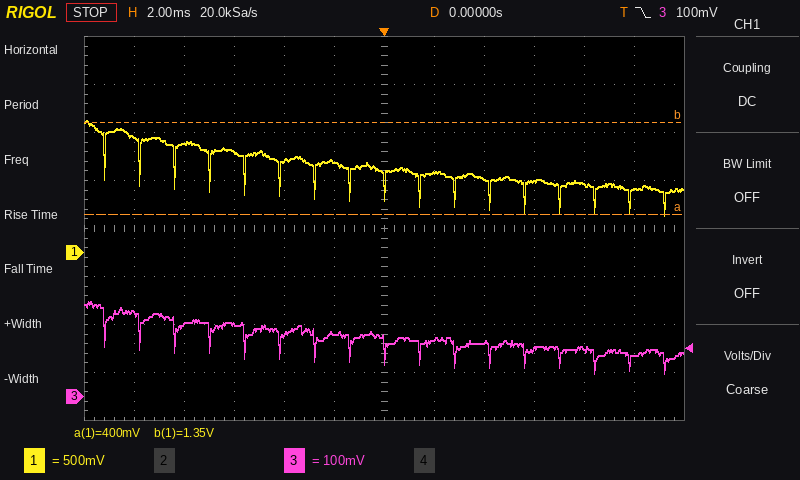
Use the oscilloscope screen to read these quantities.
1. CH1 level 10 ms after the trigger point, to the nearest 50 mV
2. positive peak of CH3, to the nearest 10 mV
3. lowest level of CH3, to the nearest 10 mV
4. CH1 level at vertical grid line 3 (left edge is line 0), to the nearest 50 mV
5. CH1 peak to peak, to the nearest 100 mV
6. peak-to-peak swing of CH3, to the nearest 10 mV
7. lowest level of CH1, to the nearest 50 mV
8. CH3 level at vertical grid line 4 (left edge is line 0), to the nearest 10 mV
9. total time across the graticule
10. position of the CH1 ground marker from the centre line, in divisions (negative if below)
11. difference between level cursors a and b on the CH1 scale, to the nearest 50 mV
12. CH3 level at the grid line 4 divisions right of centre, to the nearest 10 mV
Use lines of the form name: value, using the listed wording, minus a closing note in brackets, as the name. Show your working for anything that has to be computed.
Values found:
CH1 level 10 ms after the trigger point, to the nearest 50 mV: 650 mV
positive peak of CH3, to the nearest 10 mV: 200 mV
lowest level of CH3, to the nearest 10 mV: 50 mV
CH1 level at vertical grid line 3 (left edge is line 0), to the nearest 50 mV: 1.05 V
CH1 peak to peak, to the nearest 100 mV: 1.00 V
peak-to-peak swing of CH3, to the nearest 10 mV: 200 mV − (50 mV) = 150 mV
lowest level of CH1, to the nearest 50 mV: 400 mV
CH3 level at vertical grid line 4 (left edge is line 0), to the nearest 10 mV: 130 mV
total time across the graticule: 24 ms
position of the CH1 ground marker from the centre line, in divisions: -0.5 div
difference between level cursors a and b on the CH1 scale, to the nearest 50 mV: 950 mV
CH3 level at the grid line 4 divisions right of centre, to the nearest 10 mV: 100 mV
